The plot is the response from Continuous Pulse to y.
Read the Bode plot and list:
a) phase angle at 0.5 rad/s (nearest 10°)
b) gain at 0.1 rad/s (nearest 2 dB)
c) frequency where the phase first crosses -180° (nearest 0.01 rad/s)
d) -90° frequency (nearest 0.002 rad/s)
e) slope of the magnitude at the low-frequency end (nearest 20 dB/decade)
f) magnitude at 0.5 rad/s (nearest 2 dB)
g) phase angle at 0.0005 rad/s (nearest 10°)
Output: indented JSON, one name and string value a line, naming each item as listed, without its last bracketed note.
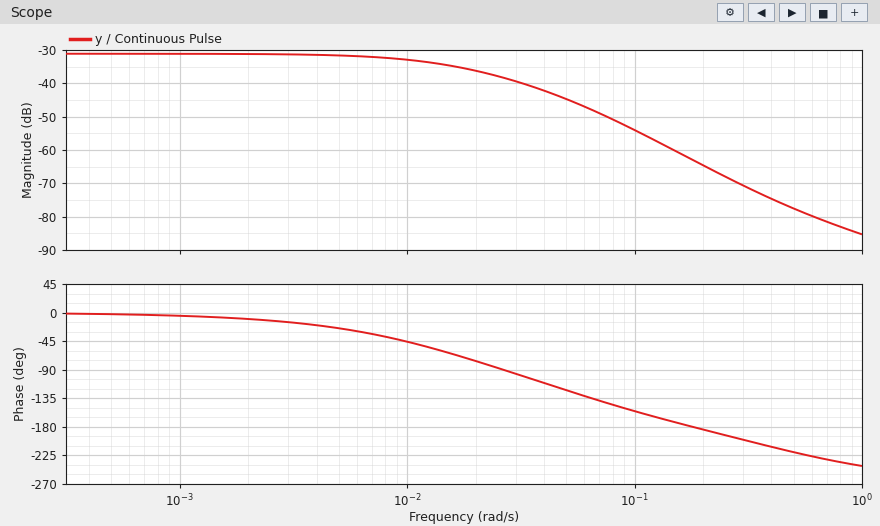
{
  "phase angle at 0.5 rad/s": "-220°",
  "gain at 0.1 rad/s": "-54 dB",
  "frequency where the phase first crosses -180°": "0.18 rad/s",
  "-90° frequency": "0.026 rad/s",
  "slope of the magnitude at the low-frequency end": "0 dB/decade",
  "magnitude at 0.5 rad/s": "-78 dB",
  "phase angle at 0.0005 rad/s": "0°"
}
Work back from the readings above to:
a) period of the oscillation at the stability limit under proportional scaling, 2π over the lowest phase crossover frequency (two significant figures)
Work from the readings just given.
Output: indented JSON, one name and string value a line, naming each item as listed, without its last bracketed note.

{
  "period of the oscillation at the stability limit under proportional scaling, 2π over the lowest phase crossover frequency": "35 s"
}
